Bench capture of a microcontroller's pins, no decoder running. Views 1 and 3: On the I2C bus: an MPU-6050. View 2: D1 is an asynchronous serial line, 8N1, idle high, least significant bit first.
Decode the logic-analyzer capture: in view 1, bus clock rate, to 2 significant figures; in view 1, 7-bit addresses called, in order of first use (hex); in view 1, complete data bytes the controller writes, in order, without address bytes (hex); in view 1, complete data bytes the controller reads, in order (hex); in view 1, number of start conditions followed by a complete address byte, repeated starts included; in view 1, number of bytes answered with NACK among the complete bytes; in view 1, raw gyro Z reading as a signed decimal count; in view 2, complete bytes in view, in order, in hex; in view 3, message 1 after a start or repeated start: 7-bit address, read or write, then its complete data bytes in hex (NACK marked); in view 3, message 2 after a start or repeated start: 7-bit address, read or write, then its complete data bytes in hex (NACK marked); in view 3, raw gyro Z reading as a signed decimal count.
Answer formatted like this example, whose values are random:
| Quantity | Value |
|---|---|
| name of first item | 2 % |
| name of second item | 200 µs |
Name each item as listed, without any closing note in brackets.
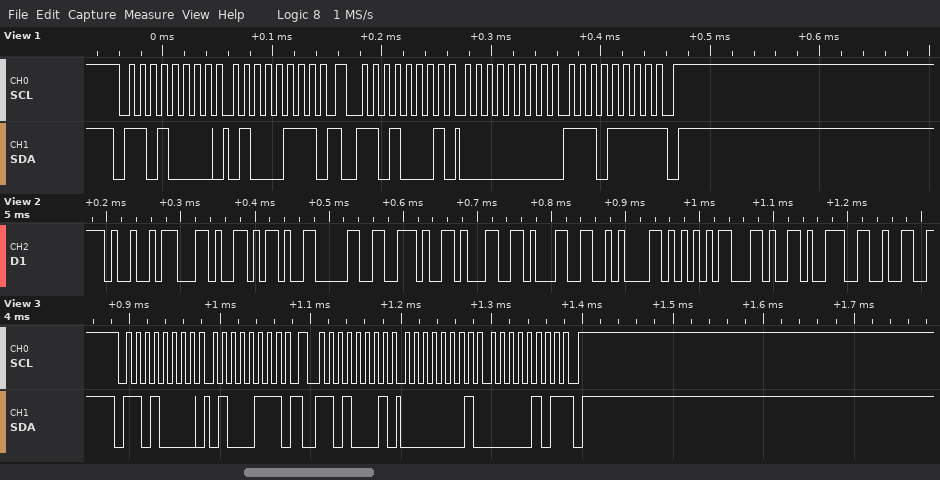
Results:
| Quantity | Value |
|---|---|
| in view 1, bus clock rate, to 2 significant figures | 100 kHz |
| in view 1, 7-bit addresses called, in order of first use | 0x68 |
| in view 1, complete data bytes the controller writes, in order, without address bytes | 47 |
| in view 1, complete data bytes the controller reads, in order | 00 EF |
| in view 1, number of start conditions followed by a complete address byte, repeated starts included | 2 |
| in view 1, number of bytes answered with NACK among the complete bytes | 1 |
| in view 1, raw gyro Z reading as a signed decimal count | 239 |
| in view 2, complete bytes in view, in order, in hex | 0x49 0x2C 0x2D 0x30 0x2E 0x31 0x31 0x0A 0x55 0x2C 0x39 0x32 |
| in view 3, message 1 after a start or repeated start: 7-bit address, read or write, then its complete data bytes in hex | 0x68 write: 47 |
| in view 3, message 2 after a start or repeated start: 7-bit address, read or write, then its complete data bytes in hex | 0x68 read: 01 05 NACK |
| in view 3, raw gyro Z reading as a signed decimal count | 261 |
